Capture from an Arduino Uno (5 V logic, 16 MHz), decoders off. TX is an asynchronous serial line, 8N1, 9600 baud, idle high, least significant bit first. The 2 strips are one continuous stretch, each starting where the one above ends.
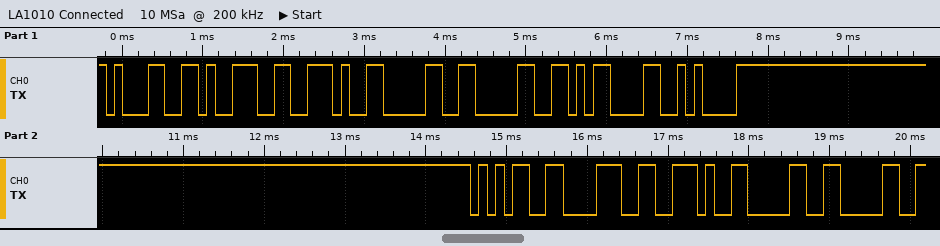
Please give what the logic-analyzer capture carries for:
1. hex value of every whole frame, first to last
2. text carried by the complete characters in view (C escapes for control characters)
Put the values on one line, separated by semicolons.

0x31 0x39 0x2E 0x30 0x30 0x0D 0x0A 0x35 0x38 0x2E 0x30 0x30; "19.00\r\n58.00"
